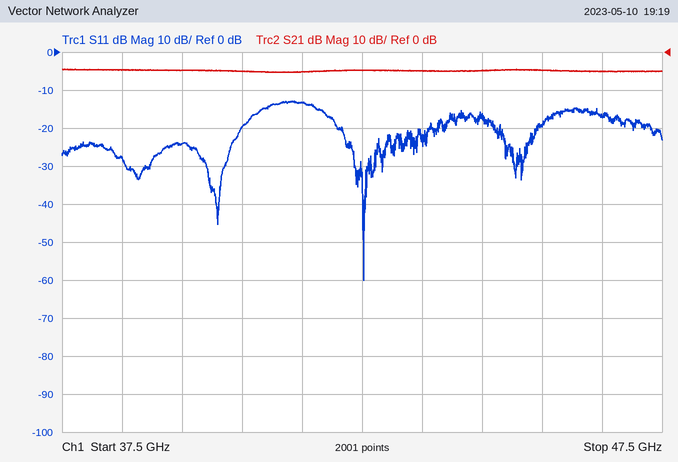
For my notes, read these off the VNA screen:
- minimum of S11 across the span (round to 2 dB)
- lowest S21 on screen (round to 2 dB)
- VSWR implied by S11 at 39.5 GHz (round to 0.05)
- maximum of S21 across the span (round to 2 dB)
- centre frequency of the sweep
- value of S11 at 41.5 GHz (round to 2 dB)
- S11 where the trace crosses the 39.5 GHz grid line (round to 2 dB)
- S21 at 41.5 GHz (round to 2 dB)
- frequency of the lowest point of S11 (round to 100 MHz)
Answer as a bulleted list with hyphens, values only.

- -60 dB
- -6 dB
- 1.15
- -4 dB
- 42.5 GHz
- -14 dB
- -24 dB
- -6 dB
- 42.5 GHz
